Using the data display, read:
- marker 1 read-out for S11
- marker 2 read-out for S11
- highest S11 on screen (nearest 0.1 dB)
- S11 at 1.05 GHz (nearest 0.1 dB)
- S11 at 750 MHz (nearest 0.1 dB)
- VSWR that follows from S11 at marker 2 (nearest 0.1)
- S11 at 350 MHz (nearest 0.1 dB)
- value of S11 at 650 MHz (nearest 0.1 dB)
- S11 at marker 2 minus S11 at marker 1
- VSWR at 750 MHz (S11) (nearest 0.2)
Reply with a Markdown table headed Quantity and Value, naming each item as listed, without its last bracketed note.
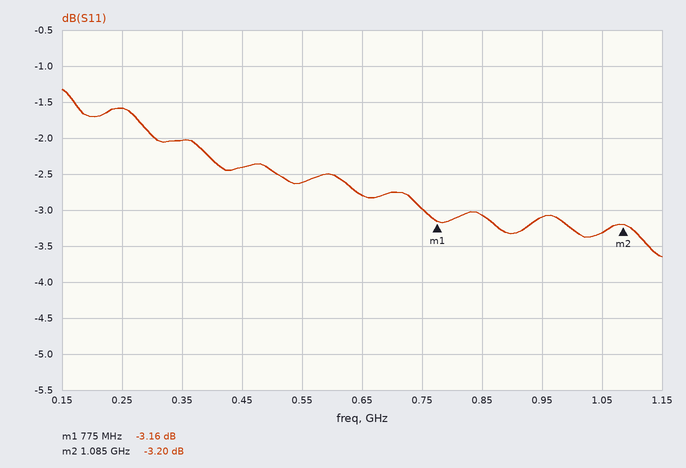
| Quantity | Value |
|---|---|
| marker 1 read-out for S11 | -3.16 dB |
| marker 2 read-out for S11 | -3.20 dB |
| highest S11 on screen | -1.3 dB |
| S11 at 1.05 GHz | -3.3 dB |
| S11 at 750 MHz | -3.0 dB |
| VSWR that follows from S11 at marker 2 | 5.5 |
| S11 at 350 MHz | -2.0 dB |
| value of S11 at 650 MHz | -2.8 dB |
| S11 at marker 2 minus S11 at marker 1 | -0.04 dB |
| VSWR at 750 MHz (S11) | 5.8 |
